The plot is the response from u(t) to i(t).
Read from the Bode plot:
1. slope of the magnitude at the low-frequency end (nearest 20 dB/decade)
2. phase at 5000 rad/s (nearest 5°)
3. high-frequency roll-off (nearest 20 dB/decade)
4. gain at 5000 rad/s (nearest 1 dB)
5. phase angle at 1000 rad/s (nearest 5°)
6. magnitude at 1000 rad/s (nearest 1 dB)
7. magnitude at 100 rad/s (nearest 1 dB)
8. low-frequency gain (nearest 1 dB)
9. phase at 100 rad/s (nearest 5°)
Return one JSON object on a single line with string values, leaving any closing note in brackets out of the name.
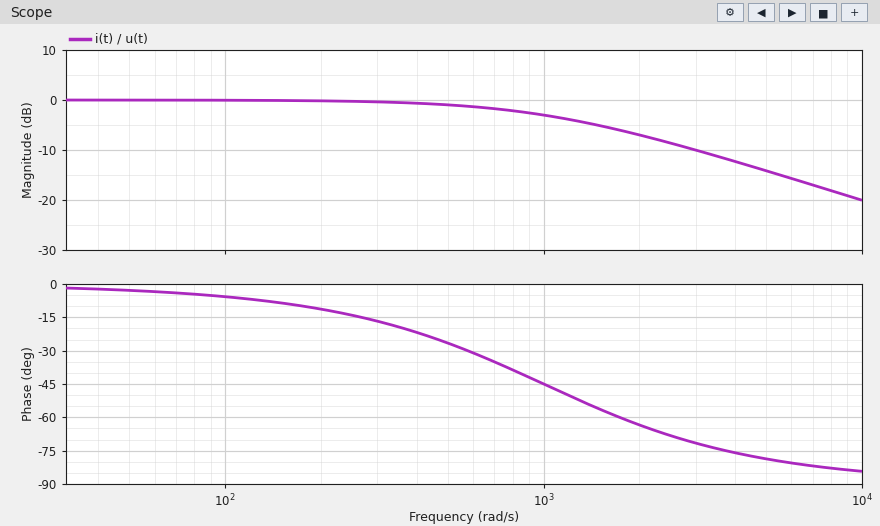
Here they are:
{"slope of the magnitude at the low-frequency end": "0 dB/decade", "phase at 5000 rad/s": "-80°", "high-frequency roll-off": "-20 dB/decade", "gain at 5000 rad/s": "-14 dB", "phase angle at 1000 rad/s": "-45°", "magnitude at 1000 rad/s": "-3 dB", "magnitude at 100 rad/s": "0 dB", "low-frequency gain": "0 dB", "phase at 100 rad/s": "-5°"}
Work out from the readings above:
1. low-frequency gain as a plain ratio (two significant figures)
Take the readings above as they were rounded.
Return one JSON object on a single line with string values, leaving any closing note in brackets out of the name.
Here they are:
{"low-frequency gain as a plain ratio": "1.0"}
